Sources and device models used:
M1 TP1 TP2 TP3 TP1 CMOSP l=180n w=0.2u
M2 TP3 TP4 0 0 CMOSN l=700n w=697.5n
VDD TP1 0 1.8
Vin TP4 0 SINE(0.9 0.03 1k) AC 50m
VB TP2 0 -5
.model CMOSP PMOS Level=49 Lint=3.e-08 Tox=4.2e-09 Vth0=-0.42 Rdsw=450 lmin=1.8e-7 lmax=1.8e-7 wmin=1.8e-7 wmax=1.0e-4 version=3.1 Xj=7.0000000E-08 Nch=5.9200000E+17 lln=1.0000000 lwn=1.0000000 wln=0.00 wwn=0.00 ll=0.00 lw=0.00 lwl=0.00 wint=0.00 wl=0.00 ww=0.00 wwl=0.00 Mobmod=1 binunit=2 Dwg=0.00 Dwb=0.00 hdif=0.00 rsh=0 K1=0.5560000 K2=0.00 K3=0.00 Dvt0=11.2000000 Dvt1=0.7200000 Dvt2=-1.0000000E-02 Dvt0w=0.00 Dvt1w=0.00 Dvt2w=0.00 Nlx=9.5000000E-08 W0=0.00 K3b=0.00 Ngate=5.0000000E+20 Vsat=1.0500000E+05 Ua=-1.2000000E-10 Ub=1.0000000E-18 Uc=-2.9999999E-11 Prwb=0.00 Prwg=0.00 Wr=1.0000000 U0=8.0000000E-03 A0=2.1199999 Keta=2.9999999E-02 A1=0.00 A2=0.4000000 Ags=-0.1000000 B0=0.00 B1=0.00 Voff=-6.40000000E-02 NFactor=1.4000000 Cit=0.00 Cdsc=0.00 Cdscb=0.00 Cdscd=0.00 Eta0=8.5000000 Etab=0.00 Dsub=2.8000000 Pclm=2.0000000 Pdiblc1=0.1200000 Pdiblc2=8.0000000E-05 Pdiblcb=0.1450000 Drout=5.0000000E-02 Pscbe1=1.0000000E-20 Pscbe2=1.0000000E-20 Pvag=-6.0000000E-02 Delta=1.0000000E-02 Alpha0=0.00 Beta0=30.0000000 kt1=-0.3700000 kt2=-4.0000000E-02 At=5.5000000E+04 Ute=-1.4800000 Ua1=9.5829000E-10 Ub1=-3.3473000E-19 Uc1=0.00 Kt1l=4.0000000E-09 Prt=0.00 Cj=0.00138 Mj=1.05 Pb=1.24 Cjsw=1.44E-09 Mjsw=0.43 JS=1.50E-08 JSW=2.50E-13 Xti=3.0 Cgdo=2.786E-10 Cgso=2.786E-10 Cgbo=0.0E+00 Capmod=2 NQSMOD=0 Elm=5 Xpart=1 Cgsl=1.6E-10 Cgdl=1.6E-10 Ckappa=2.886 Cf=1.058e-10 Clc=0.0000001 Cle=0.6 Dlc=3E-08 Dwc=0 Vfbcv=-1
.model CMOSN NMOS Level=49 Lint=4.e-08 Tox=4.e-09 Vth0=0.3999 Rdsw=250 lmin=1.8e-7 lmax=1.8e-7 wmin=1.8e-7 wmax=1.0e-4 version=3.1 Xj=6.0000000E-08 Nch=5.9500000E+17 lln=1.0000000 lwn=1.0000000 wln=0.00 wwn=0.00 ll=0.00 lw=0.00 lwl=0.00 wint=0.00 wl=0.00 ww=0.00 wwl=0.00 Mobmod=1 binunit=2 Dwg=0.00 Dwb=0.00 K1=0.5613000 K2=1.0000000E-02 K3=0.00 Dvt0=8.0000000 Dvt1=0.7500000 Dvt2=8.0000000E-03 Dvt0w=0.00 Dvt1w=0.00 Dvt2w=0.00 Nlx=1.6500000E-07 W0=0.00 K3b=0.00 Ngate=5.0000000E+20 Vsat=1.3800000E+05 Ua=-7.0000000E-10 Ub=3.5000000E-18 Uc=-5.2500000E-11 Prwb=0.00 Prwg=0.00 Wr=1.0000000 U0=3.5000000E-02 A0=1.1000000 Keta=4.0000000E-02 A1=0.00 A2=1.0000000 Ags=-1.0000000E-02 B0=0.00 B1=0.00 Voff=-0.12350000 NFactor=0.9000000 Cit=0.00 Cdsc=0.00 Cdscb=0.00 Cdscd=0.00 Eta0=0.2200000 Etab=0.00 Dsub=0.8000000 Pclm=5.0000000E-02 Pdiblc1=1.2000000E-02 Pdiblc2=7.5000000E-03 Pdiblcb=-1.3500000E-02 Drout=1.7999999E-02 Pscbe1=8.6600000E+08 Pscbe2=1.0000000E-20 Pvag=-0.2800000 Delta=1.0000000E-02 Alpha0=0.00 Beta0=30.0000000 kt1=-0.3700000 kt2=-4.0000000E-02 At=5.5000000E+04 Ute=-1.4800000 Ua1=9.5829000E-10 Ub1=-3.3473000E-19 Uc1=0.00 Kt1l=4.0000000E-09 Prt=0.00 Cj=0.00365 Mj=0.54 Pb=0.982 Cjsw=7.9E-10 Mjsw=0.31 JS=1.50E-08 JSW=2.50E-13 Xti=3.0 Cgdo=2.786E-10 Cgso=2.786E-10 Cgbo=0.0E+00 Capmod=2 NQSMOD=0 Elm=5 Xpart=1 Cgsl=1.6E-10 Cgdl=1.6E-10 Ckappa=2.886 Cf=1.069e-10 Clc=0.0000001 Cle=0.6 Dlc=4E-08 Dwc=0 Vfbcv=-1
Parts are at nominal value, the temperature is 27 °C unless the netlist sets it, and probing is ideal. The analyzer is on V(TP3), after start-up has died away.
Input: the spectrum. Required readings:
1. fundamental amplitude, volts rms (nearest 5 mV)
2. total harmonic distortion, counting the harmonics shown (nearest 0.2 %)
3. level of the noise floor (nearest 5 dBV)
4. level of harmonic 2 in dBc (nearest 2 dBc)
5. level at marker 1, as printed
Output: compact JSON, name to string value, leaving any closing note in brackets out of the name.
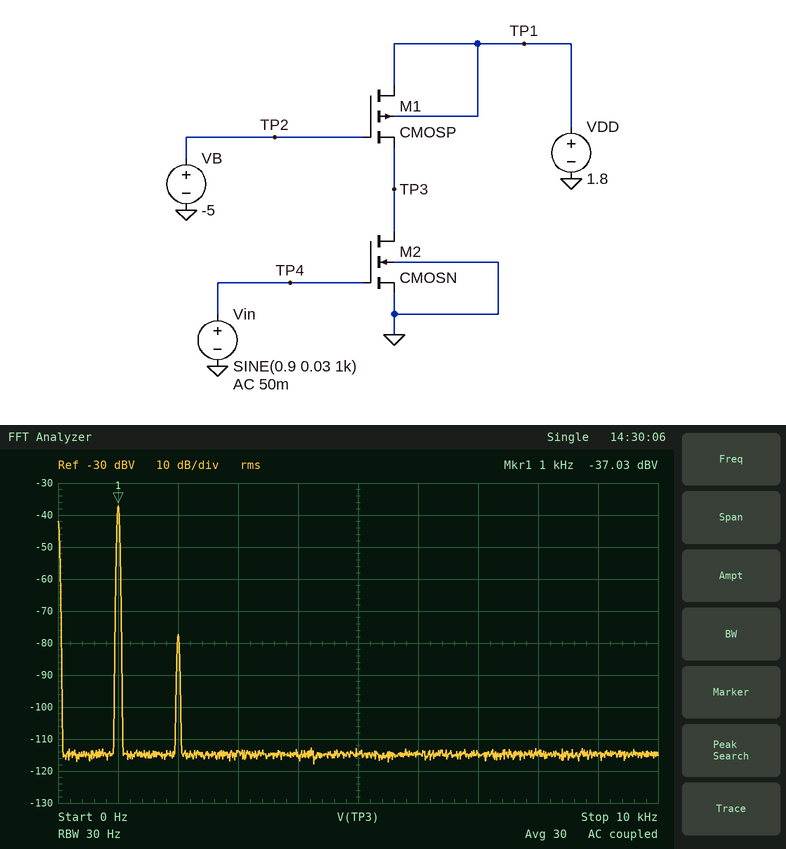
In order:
{"fundamental amplitude, volts rms": "15 mV", "total harmonic distortion, counting the harmonics shown": "1.0 %", "level of the noise floor": "-115 dBV", "level of harmonic 2 in dBc": "-40 dBc", "level at marker 1, as printed": "-37.03 dBV"}
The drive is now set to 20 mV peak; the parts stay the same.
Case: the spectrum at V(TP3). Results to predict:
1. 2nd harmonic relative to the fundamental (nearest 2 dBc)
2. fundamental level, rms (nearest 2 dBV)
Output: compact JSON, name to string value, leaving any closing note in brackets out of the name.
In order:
{"2nd harmonic relative to the fundamental": "-44 dBc", "fundamental level, rms": "-40 dBV"}
